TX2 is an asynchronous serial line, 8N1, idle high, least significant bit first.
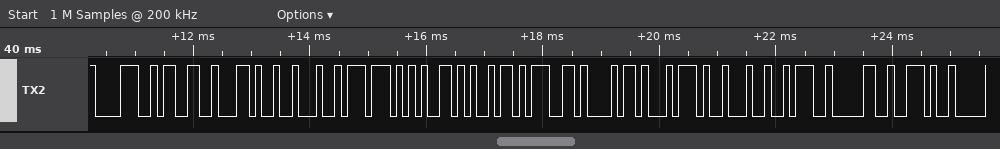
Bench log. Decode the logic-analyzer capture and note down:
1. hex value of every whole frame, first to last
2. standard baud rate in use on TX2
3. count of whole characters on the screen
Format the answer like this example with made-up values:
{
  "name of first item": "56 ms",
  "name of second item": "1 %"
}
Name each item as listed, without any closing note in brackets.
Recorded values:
{
  "hex value of every whole frame, first to last": "0x38 0x33 0x2C 0x22 0x77 0x65 0x69 0x67 0x68 0x74 0x22 0x3A 0x30 0x2E",
  "standard baud rate in use on TX2": "9600 baud",
  "count of whole characters on the screen": "14"
}
